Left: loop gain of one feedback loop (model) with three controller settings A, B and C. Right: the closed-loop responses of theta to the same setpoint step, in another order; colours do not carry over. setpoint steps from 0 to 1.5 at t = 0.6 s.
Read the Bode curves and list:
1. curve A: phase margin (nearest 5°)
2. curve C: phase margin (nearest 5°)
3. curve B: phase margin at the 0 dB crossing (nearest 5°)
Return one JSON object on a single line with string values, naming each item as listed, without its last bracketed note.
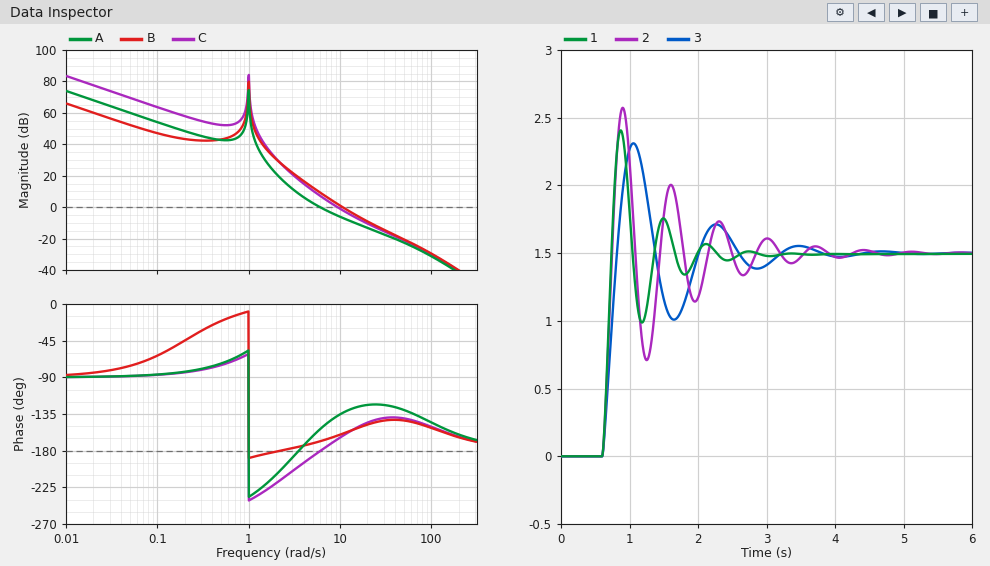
{"curve A: phase margin": "25°", "curve C: phase margin": "15°", "curve B: phase margin at the 0 dB crossing": "20°"}
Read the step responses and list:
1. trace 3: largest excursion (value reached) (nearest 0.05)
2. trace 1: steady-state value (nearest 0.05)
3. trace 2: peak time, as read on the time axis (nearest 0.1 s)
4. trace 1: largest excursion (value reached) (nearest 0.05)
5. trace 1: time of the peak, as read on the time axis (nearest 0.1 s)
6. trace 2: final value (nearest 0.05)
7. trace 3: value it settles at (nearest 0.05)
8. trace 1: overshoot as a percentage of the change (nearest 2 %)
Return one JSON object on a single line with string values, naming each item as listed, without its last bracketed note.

{"trace 3: largest excursion (value reached)": "2.30", "trace 1: steady-state value": "1.50", "trace 2: peak time, as read on the time axis": "0.9 s", "trace 1: largest excursion (value reached)": "2.40", "trace 1: time of the peak, as read on the time axis": "0.9 s", "trace 2: final value": "1.50", "trace 3: value it settles at": "1.50", "trace 1: overshoot as a percentage of the change": "60 %"}
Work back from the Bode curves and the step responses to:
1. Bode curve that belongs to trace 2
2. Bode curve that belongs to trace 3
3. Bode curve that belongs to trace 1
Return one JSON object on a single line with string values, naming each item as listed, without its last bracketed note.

{"Bode curve that belongs to trace 2": "C", "Bode curve that belongs to trace 3": "A", "Bode curve that belongs to trace 1": "B"}
